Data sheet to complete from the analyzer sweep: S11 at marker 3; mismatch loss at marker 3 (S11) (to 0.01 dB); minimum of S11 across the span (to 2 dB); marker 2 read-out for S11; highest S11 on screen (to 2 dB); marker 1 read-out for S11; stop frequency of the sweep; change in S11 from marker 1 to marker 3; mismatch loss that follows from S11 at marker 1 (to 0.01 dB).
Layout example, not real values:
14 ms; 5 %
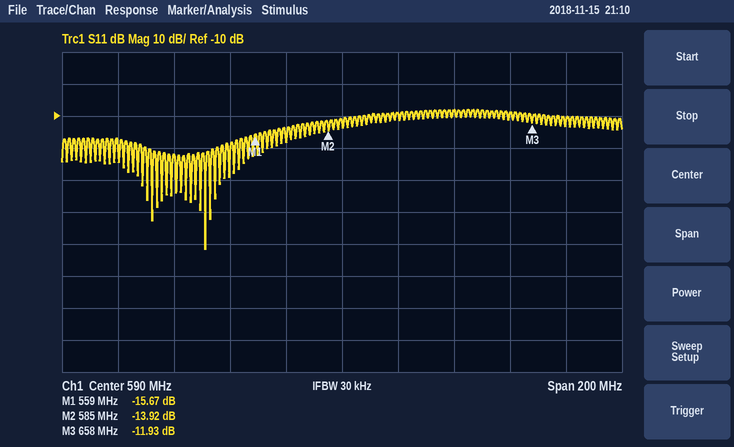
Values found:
-11.93 dB; 0.29 dB; -52 dB; -13.92 dB; -8 dB; -15.67 dB; 690 MHz; 3.74 dB; 0.12 dB
